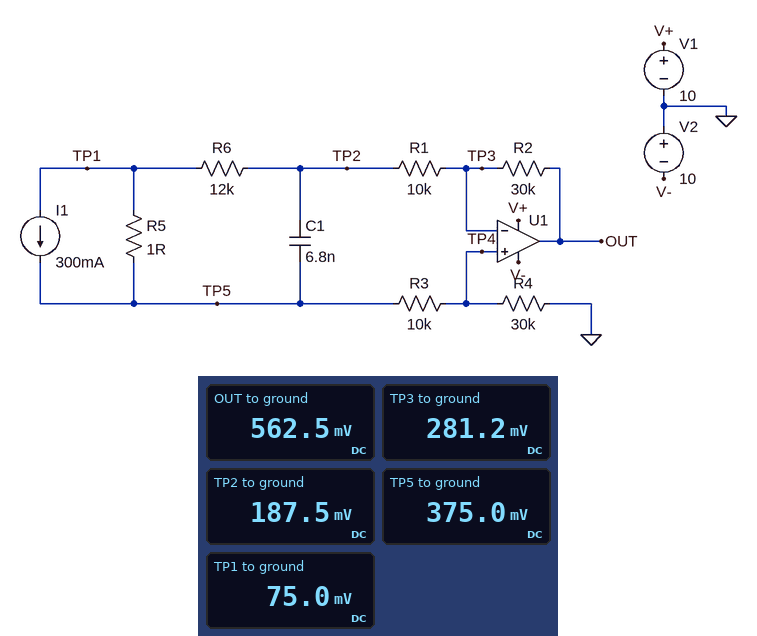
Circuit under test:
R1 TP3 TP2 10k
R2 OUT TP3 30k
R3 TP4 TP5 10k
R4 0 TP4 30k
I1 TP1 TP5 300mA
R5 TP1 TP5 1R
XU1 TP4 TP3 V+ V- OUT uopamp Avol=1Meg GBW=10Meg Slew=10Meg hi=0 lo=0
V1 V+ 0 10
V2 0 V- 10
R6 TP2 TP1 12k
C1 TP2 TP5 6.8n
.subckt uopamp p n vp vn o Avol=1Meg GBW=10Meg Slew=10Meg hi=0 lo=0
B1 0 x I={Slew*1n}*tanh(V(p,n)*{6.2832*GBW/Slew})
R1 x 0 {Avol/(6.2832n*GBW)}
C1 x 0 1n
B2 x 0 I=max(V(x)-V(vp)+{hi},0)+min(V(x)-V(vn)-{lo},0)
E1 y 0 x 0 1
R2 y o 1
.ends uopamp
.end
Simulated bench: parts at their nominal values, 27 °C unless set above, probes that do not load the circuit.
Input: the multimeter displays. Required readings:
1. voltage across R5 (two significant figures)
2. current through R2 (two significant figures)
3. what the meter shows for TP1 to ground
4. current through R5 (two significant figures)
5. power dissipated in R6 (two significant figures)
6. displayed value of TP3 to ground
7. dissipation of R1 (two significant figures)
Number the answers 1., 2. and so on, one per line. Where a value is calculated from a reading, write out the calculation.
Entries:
1. 375 mV - 75 mV = 300 mV
2. (562.5 mV - 281.2 mV) / 30 kΩ = 9.4 µA
3. 75.0 mV
4. (375 mV - 75 mV) / 1 Ω = 300 mA
5. (187.5 mV - 75 mV)^2 / 12 kΩ = 1.1 µW
6. 281.2 mV
7. (281.2 mV - 187.5 mV)^2 / 10 kΩ = 880 nW
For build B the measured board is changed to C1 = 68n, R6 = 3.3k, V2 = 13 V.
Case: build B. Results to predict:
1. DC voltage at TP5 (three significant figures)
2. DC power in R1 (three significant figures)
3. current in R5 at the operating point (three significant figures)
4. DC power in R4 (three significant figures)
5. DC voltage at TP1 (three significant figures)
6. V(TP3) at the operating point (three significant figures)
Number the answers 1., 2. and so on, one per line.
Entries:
1. 515 mV
2. 1.66 µW
3. 300 mA
4. 4.97 µW
5. 215 mV
6. 386 mV
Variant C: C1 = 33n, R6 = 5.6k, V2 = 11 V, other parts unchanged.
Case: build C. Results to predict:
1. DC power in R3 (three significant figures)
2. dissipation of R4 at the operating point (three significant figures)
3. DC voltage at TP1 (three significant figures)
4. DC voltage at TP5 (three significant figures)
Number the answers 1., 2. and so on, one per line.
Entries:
1. 1.37 µW
2. 4.12 µW
3. 169 mV
4. 469 mV
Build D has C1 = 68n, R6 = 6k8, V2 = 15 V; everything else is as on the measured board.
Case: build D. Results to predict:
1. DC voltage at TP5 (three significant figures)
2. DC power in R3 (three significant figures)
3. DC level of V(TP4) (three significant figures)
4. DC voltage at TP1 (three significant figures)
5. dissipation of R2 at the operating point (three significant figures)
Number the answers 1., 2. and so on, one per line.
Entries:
1. 448 mV
2. 1.25 µW
3. 336 mV
4. 148 mV
5. 3.76 µW
